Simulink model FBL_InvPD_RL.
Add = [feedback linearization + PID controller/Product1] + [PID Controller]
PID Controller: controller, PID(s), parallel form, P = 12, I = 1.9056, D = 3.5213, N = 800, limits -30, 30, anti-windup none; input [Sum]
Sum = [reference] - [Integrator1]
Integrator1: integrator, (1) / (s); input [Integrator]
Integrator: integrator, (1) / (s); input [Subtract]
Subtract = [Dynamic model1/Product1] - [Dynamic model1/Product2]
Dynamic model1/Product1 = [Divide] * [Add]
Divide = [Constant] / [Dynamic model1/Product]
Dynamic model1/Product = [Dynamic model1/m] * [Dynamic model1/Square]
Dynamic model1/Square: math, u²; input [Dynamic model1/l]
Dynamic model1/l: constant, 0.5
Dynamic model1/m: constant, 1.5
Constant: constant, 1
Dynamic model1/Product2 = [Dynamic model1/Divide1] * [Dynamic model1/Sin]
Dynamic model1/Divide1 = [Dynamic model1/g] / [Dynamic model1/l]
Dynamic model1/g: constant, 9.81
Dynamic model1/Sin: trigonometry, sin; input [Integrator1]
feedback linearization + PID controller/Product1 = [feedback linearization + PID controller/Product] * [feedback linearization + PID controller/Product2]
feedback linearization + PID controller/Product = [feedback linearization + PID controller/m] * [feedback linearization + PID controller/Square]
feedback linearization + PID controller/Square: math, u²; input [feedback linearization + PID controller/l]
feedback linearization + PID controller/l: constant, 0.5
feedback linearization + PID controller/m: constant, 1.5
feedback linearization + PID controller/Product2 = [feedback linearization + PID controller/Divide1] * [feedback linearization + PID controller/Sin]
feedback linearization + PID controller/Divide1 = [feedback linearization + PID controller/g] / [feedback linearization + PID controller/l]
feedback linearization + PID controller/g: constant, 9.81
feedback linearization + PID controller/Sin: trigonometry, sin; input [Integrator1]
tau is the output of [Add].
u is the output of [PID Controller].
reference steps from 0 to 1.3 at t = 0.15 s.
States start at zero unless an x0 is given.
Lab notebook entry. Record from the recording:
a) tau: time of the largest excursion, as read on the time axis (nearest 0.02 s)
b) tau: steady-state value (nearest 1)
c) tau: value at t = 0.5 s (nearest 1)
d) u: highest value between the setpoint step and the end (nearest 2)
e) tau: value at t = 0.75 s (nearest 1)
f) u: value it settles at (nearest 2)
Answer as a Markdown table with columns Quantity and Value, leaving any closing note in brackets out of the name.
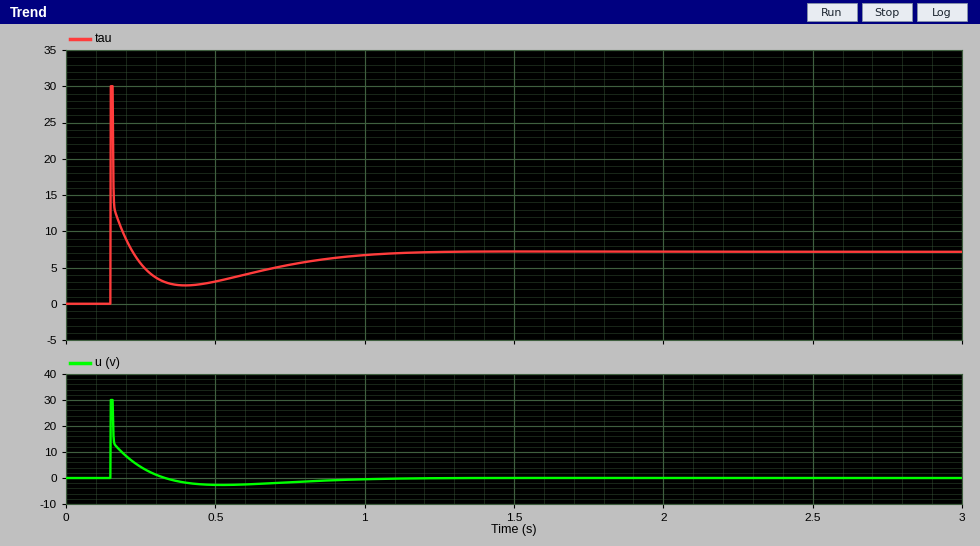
| Quantity | Value |
|---|---|
| tau: time of the largest excursion, as read on the time axis | 0.16 s |
| tau: steady-state value | 7 |
| tau: value at t = 0.5 s | 3 |
| u: highest value between the setpoint step and the end | 30 |
| tau: value at t = 0.75 s | 5 |
| u: value it settles at | 0 |
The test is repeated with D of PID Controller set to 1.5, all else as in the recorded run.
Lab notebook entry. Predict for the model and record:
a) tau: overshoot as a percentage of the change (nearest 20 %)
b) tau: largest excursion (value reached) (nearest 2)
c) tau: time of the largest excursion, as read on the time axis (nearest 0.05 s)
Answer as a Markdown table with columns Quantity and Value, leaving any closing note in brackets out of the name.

| Quantity | Value |
|---|---|
| tau: overshoot as a percentage of the change | 320 % |
| tau: largest excursion (value reached) | 30 |
| tau: time of the largest excursion, as read on the time axis | 0.15 s |
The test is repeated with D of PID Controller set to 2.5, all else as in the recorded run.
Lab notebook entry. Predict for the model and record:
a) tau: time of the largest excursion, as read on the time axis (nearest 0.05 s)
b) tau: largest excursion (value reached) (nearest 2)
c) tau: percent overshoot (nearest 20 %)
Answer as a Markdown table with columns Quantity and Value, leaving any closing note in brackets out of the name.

| Quantity | Value |
|---|---|
| tau: time of the largest excursion, as read on the time axis | 0.15 s |
| tau: largest excursion (value reached) | 30 |
| tau: percent overshoot | 320 % |
